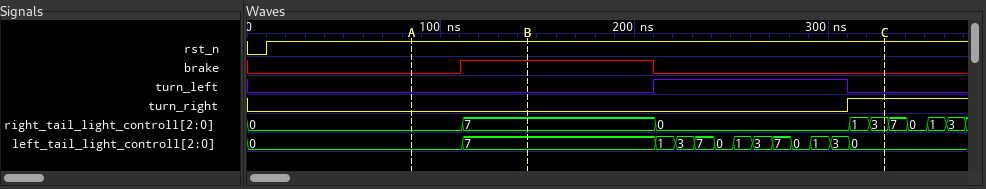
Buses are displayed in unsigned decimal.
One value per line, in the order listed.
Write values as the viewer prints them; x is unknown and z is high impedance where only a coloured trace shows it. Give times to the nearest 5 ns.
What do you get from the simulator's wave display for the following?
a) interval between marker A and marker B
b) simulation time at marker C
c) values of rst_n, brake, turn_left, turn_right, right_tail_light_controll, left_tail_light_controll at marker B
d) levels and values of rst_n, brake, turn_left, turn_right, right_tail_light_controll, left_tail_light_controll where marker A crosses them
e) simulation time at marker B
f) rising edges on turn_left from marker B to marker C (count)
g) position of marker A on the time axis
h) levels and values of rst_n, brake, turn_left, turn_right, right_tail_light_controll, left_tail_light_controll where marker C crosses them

60 ns
330 ns
rst_n=1, brake=1, turn_left=0, turn_right=0, right_tail_light_controll=7, left_tail_light_controll=7
rst_n=1, brake=0, turn_left=0, turn_right=0, right_tail_light_controll=0, left_tail_light_controll=0
145 ns
1
85 ns
rst_n=1, brake=0, turn_left=0, turn_right=1, right_tail_light_controll=3, left_tail_light_controll=0
